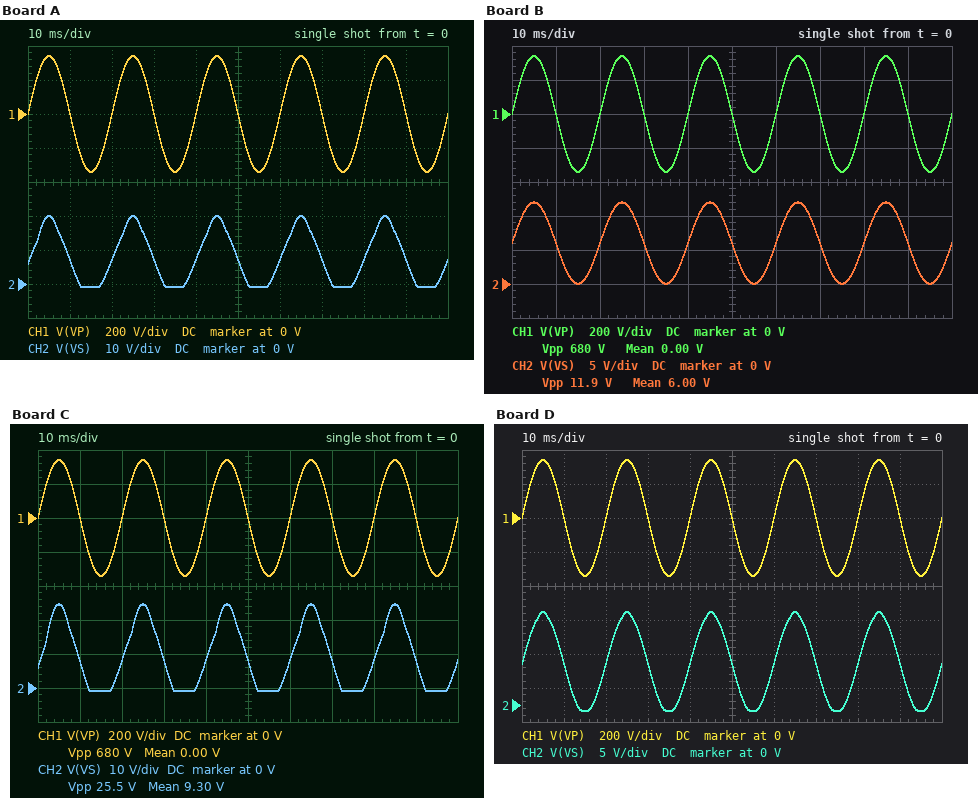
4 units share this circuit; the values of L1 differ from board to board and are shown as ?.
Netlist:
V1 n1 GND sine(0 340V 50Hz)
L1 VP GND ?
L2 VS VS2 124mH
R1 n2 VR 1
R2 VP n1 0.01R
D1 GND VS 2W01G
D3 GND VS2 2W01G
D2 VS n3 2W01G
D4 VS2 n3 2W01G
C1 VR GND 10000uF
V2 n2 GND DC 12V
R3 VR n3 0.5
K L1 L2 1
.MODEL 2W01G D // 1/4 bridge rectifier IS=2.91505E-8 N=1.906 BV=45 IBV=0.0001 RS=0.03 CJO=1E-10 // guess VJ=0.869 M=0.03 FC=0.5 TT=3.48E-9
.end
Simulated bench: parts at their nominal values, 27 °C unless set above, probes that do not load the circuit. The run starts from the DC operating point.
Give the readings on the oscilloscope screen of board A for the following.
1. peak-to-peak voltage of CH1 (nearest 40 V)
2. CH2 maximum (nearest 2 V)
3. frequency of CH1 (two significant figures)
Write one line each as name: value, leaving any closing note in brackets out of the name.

peak-to-peak voltage of CH1: 680 V
CH2 maximum: 20 V
frequency of CH1: 50 Hz
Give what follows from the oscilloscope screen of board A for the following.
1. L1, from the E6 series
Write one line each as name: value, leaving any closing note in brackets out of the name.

L1, from the E6 series: 33 H
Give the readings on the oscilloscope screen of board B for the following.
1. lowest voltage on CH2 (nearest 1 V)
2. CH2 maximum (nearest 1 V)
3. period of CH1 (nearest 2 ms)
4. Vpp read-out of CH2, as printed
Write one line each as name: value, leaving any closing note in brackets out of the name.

lowest voltage on CH2: 0 V
CH2 maximum: 12 V
period of CH1: 20 ms
Vpp read-out of CH2, as printed: 11.9 V
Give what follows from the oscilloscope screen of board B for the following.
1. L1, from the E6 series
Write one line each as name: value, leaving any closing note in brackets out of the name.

L1, from the E6 series: 100 H
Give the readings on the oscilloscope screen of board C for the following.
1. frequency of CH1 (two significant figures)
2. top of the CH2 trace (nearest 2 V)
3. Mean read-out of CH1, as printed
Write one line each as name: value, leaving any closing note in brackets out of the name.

frequency of CH1: 50 Hz
top of the CH2 trace: 24 V
Mean read-out of CH1, as printed: 0.00 V
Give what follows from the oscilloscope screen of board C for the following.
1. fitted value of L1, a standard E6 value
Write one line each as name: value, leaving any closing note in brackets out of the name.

fitted value of L1, a standard E6 value: 22 H
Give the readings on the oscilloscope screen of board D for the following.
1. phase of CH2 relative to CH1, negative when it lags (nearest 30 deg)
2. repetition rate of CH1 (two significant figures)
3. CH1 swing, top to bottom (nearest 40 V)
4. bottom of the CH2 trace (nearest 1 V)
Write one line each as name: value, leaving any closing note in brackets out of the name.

phase of CH2 relative to CH1, negative when it lags: 0 deg
repetition rate of CH1: 50 Hz
CH1 swing, top to bottom: 680 V
bottom of the CH2 trace: -1 V
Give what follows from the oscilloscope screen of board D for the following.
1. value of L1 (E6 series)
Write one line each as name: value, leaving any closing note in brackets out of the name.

value of L1: 68 H
